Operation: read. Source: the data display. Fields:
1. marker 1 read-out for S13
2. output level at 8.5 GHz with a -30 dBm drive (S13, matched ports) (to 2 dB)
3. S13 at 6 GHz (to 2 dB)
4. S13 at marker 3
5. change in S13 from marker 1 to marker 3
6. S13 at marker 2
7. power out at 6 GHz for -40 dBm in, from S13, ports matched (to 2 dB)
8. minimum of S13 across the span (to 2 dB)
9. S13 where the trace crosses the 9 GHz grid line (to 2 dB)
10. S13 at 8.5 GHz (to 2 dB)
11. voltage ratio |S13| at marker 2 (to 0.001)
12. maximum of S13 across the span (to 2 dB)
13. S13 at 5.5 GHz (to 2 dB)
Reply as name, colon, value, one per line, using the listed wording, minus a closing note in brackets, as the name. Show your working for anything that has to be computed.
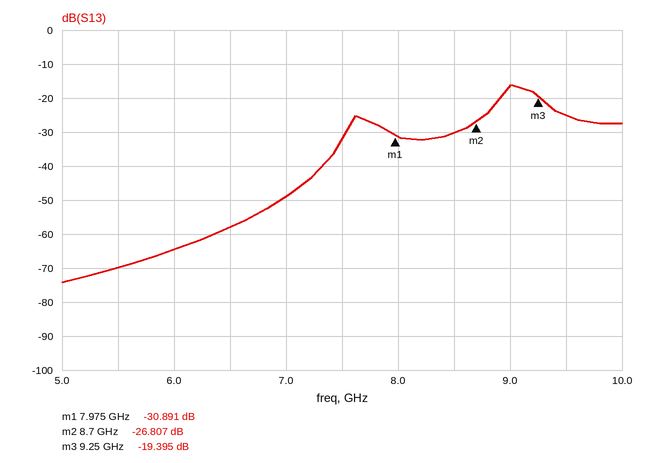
marker 1 read-out for S13: -30.891 dB
output level at 8.5 GHz with a -30 dBm drive (S13, matched ports): -30 dBm + (-30 dB) = -60 dBm
S13 at 6 GHz: -64 dB
S13 at marker 3: -19.395 dB
change in S13 from marker 1 to marker 3: -19.395 − (-30.891) = 11.496 dB
S13 at marker 2: -26.807 dB
power out at 6 GHz for -40 dBm in, from S13, ports matched: -40 dBm + (-64 dB) = -104 dBm
minimum of S13 across the span: -74 dB
S13 where the trace crosses the 9 GHz grid line: -16 dB
S13 at 8.5 GHz: -30 dB
voltage ratio |S13| at marker 2: 10^(-26.807/20) ≈ 0.046
maximum of S13 across the span: -16 dB
S13 at 5.5 GHz: -70 dB
